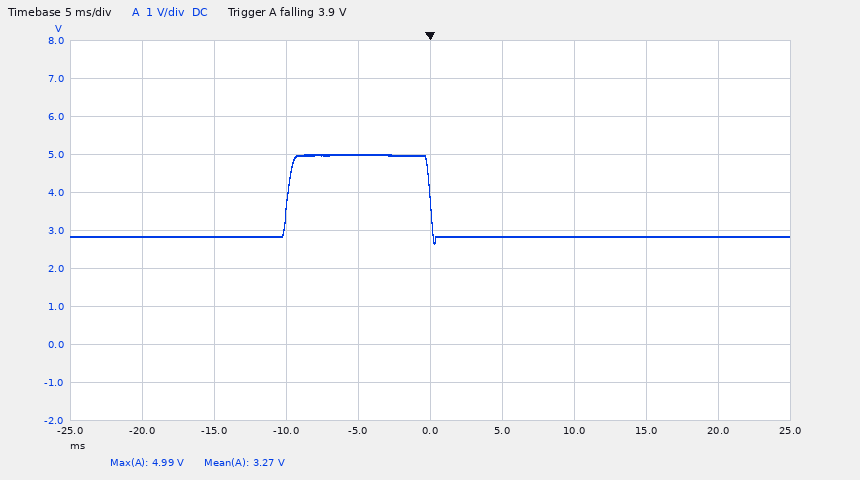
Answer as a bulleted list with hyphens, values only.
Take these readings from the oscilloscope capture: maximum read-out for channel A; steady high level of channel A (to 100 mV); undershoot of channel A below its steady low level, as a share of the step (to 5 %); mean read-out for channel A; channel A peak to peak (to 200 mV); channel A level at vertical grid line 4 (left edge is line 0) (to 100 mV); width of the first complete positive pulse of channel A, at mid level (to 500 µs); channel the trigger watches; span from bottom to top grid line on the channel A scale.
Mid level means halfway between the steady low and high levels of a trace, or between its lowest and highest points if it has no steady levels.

- 4.99 V
- 5.0 V
- 10 %
- 3.27 V
- 2.4 V
- 5.0 V
- 10.0 ms
- channel A
- 10 V
